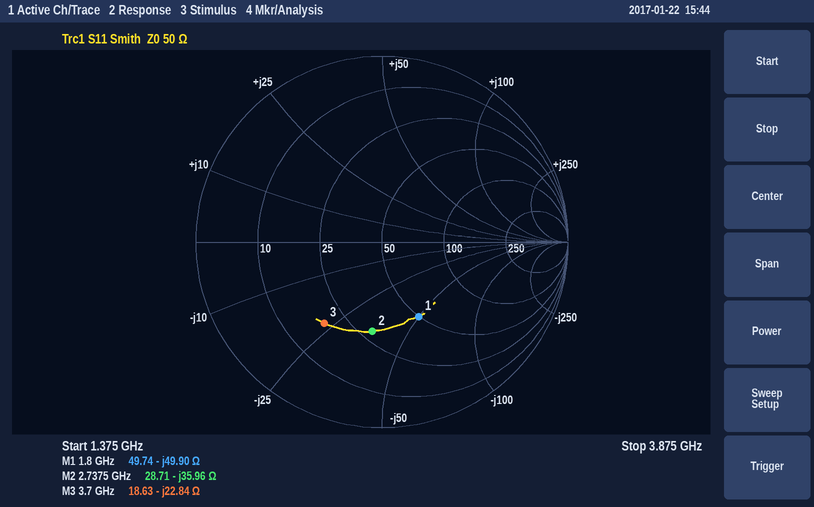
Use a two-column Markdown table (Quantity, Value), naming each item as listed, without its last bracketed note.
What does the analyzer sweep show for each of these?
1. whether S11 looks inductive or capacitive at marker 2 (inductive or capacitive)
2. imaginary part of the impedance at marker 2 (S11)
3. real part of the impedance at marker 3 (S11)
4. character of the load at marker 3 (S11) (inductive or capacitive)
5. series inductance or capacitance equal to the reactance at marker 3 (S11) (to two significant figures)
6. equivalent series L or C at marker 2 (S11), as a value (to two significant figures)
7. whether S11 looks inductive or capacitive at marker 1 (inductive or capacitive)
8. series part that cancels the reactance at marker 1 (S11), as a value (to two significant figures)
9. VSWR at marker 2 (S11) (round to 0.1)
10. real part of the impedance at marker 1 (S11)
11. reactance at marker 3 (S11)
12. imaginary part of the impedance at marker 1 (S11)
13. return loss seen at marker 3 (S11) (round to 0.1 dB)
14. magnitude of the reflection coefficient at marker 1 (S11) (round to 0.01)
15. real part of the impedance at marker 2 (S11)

| Quantity | Value |
|---|---|
| whether S11 looks inductive or capacitive at marker 2 | capacitive |
| imaginary part of the impedance at marker 2 | -35.96 Ω |
| real part of the impedance at marker 3 | 18.63 Ω |
| character of the load at marker 3 (S11) | capacitive |
| series inductance or capacitance equal to the reactance at marker 3 (S11) | 1.9 pF |
| equivalent series L or C at marker 2 (S11), as a value | 1.6 pF |
| whether S11 looks inductive or capacitive at marker 1 | capacitive |
| series part that cancels the reactance at marker 1 (S11), as a value | 4.4 nH |
| VSWR at marker 2 (S11) | 2.9 |
| real part of the impedance at marker 1 | 49.74 Ω |
| reactance at marker 3 | -22.84 Ω |
| imaginary part of the impedance at marker 1 | -49.90 Ω |
| return loss seen at marker 3 (S11) | 5.4 dB |
| magnitude of the reflection coefficient at marker 1 (S11) | 0.45 |
| real part of the impedance at marker 2 | 28.71 Ω |
